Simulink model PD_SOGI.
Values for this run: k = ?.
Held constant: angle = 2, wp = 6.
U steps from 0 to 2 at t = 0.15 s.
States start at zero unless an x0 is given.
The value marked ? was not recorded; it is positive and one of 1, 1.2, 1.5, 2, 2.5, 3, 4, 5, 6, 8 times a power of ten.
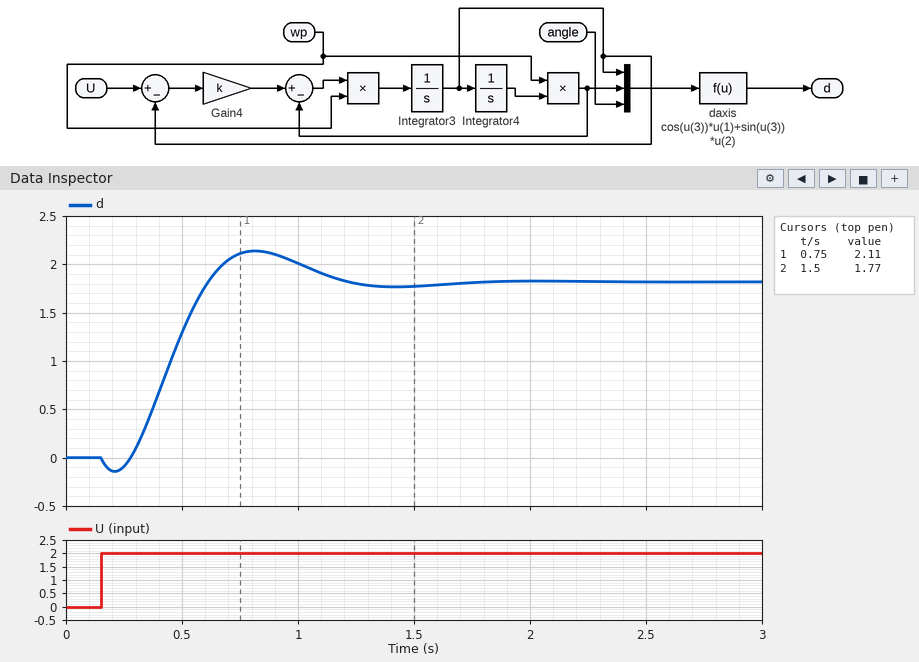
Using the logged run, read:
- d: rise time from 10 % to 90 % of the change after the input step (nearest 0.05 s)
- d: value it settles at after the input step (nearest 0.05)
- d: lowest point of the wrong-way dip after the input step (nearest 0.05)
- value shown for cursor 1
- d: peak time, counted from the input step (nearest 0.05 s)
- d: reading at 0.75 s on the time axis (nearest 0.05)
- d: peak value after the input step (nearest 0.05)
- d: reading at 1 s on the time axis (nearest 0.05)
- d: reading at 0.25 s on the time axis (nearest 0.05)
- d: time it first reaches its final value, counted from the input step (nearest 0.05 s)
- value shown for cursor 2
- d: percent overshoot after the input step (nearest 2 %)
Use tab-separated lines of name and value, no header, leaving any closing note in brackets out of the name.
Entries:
d: rise time from 10 % to 90 % of the change after the input step	0.25 s
d: value it settles at after the input step	1.80
d: lowest point of the wrong-way dip after the input step	-0.15
value shown for cursor 1	2.11
d: peak time, counted from the input step	0.65 s
d: reading at 0.75 s on the time axis	2.10
d: peak value after the input step	2.15
d: reading at 1 s on the time axis	2.00
d: reading at 0.25 s on the time axis	-0.10
d: time it first reaches its final value, counted from the input step	0.45 s
value shown for cursor 2	1.77
d: percent overshoot after the input step	18 %
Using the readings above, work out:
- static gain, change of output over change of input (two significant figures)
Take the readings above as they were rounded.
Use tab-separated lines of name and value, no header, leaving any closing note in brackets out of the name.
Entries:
static gain, change of output over change of input	0.90
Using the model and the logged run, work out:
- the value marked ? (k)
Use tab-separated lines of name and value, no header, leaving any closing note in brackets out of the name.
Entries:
the value marked ?	1
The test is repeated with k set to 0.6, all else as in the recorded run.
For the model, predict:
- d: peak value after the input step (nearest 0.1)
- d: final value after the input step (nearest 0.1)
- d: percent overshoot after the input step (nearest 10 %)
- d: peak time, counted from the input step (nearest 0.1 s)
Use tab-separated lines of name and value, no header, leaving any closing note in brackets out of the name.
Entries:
d: peak value after the input step	1.5
d: final value after the input step	1.1
d: percent overshoot after the input step	40 %
d: peak time, counted from the input step	0.6 s
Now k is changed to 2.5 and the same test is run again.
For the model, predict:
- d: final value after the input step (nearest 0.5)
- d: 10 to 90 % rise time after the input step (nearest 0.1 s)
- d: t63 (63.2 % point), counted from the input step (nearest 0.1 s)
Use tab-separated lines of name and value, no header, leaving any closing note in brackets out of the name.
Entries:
d: final value after the input step	4.5
d: 10 to 90 % rise time after the input step	0.8 s
d: t63 (63.2 % point), counted from the input step	0.5 s
